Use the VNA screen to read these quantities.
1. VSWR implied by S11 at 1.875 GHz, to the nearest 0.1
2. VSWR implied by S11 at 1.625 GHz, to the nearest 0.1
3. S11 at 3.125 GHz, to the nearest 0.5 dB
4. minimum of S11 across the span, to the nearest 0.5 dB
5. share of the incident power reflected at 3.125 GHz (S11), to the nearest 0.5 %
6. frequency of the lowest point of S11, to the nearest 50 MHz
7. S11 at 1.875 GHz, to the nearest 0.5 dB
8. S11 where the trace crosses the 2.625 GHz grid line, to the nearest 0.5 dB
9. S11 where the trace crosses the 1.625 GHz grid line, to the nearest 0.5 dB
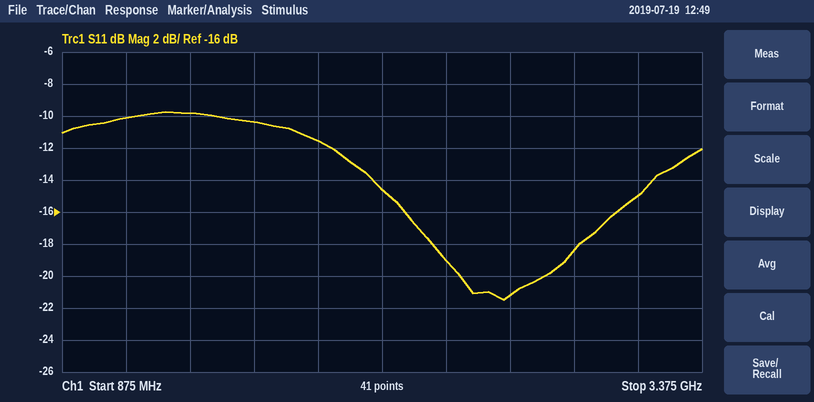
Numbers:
1.7
1.9
-15.0 dB
-21.5 dB
3.0 %
2.60 GHz
-11.5 dB
-21.0 dB
-10.5 dB
